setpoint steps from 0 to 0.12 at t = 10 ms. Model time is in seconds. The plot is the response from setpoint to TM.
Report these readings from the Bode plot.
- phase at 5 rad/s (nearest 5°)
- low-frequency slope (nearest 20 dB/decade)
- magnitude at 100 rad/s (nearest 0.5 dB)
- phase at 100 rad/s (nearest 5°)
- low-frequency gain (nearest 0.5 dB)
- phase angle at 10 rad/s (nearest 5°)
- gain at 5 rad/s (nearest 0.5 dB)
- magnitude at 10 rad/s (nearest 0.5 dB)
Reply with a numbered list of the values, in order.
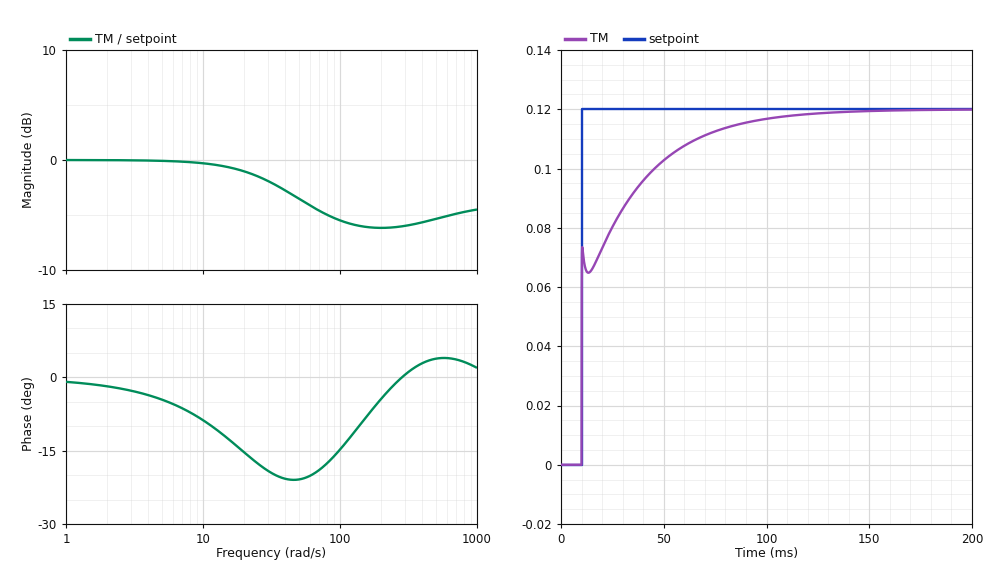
1. -5°
2. 0 dB/decade
3. -5.5 dB
4. -15°
5. 0.0 dB
6. -10°
7. 0.0 dB
8. -0.5 dB
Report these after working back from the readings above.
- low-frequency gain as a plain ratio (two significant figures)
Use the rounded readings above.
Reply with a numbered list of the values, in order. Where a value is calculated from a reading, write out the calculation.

1. 10^(0 / 20) = 1.0
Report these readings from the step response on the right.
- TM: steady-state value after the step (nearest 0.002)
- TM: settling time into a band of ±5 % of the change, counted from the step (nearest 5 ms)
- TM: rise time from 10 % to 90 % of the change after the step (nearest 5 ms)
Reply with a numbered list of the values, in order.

1. 0.120
2. 70 ms
3. 50 ms
